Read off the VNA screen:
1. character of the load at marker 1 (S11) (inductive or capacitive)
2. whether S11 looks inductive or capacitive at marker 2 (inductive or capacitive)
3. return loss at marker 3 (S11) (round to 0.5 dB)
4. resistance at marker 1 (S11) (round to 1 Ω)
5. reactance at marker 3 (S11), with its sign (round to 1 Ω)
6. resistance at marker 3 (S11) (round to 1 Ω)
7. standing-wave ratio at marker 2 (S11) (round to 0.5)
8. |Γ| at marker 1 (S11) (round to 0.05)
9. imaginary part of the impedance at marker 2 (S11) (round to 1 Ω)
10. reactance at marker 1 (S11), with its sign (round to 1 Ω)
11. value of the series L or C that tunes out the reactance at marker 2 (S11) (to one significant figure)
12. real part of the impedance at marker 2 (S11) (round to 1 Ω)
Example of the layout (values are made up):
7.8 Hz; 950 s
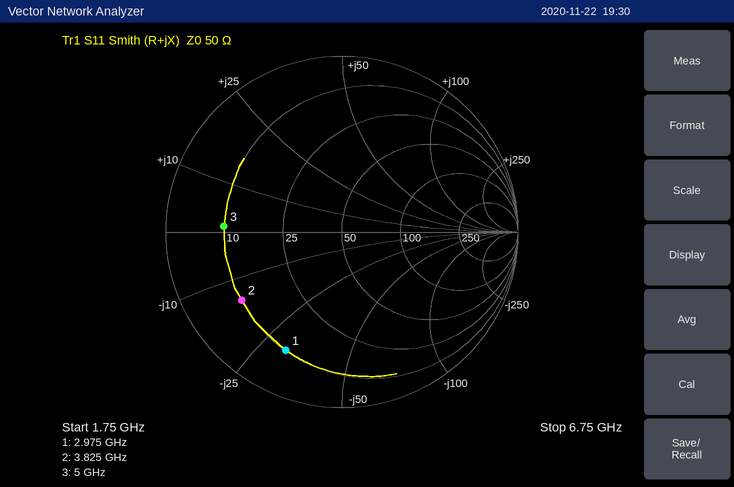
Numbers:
capacitive; capacitive; 3.5 dB; 10 Ω; +1 Ω; 10 Ω; 5.5; 0.75; -15 Ω; -31 Ω; 600 pH; 10 Ω
